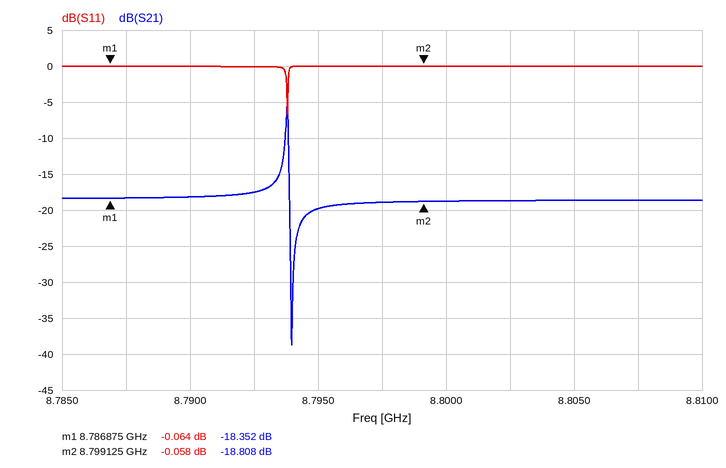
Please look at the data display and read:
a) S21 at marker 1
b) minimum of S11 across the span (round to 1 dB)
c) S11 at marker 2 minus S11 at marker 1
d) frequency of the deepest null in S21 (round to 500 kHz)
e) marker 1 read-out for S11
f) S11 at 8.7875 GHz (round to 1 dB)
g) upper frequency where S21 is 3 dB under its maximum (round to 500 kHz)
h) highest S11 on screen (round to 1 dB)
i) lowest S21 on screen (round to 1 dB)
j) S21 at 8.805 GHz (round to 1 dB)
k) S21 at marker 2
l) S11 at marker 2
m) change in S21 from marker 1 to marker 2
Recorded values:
-18.352 dB
-7 dB
0.006 dB
8.7940 GHz
-0.064 dB
0 dB
8.7940 GHz
0 dB
-39 dB
-19 dB
-18.808 dB
-0.058 dB
-0.456 dB
